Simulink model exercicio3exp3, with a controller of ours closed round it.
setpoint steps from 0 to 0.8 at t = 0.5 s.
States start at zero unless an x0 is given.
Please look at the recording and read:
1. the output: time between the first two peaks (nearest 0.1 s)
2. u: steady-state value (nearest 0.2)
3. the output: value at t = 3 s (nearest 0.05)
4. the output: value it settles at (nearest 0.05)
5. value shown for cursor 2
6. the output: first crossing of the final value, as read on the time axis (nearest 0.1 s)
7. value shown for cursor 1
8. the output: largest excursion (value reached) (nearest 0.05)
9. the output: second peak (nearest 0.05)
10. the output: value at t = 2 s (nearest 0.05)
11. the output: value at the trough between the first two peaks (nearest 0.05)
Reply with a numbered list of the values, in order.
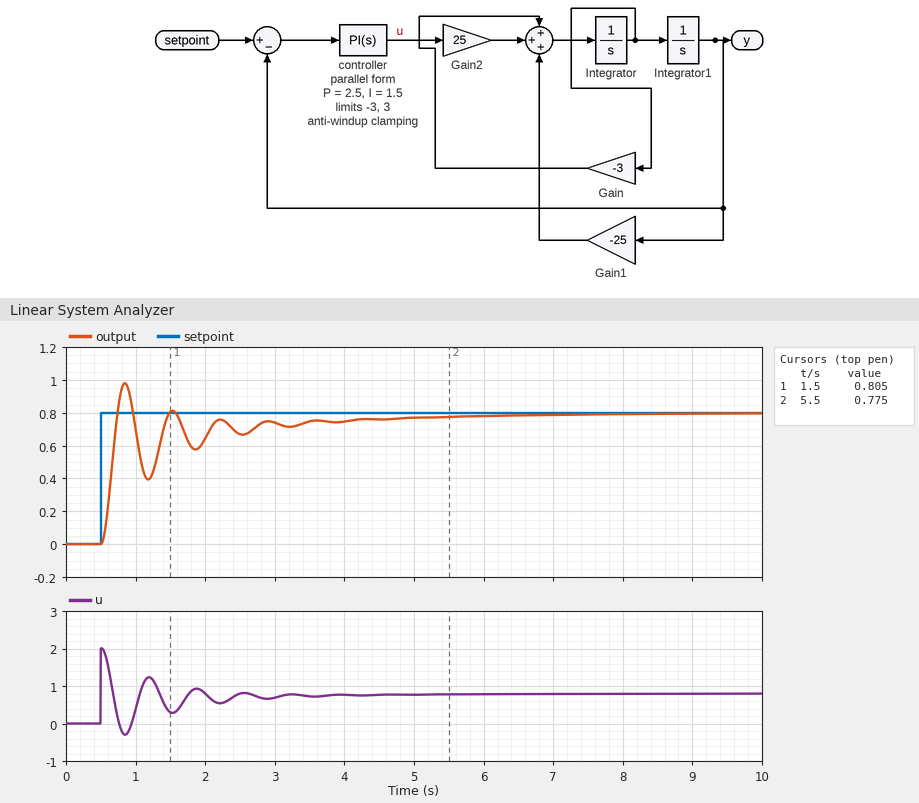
1. 0.7 s
2. 0.8
3. 0.75
4. 0.80
5. 0.775
6. 0.7 s
7. 0.805
8. 1.00
9. 0.80
10. 0.65
11. 0.40
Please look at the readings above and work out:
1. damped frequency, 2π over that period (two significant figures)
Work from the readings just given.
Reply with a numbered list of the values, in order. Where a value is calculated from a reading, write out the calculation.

1. 2π / 0.7 = 9.0 rad/s
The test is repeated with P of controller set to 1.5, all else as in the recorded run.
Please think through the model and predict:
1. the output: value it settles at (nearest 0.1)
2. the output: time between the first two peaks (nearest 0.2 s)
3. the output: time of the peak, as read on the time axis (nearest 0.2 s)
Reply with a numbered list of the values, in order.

1. 0.8
2. 0.8 s
3. 1.0 s
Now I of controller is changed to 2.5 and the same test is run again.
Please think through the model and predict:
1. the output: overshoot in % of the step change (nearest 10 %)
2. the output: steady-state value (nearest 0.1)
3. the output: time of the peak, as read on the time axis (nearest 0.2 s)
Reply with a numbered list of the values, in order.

1. 30 %
2. 0.8
3. 0.8 s
